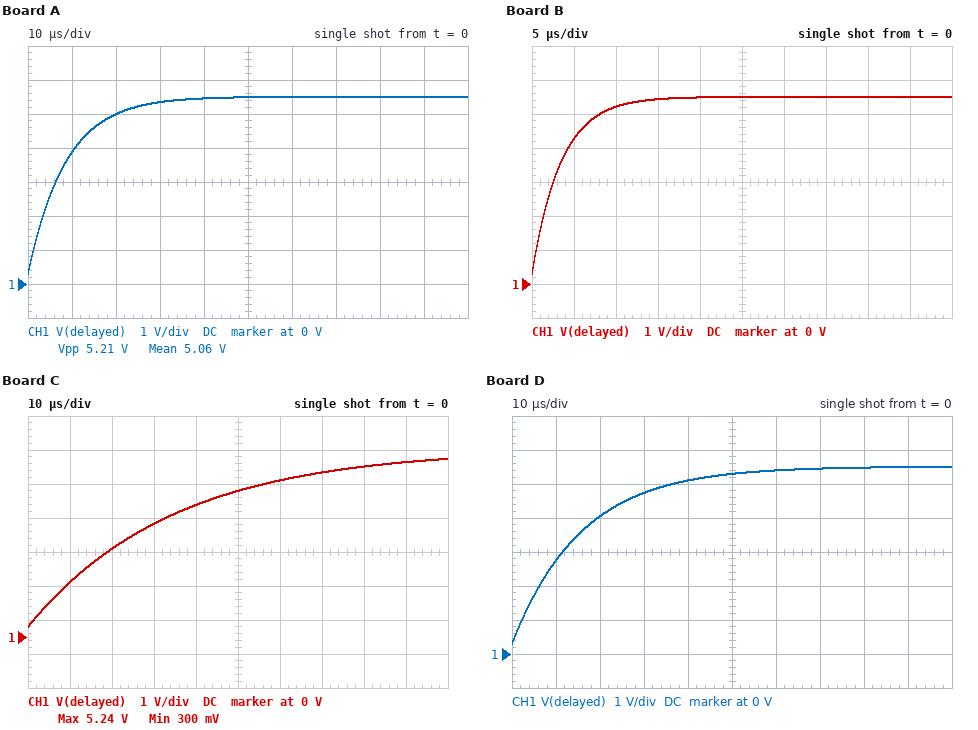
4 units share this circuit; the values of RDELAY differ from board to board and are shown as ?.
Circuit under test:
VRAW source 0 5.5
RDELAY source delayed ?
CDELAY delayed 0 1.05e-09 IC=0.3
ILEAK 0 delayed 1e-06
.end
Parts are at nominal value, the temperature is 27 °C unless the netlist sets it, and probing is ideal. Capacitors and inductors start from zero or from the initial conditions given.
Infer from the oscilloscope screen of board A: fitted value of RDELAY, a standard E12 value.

8.2 kΩ
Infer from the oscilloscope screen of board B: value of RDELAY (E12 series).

3.3 kΩ
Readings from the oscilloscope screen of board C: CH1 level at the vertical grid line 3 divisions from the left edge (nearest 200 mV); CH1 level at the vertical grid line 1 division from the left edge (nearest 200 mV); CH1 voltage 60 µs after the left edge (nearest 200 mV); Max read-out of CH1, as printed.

3.4 V
1.6 V
4.6 V
5.24 V
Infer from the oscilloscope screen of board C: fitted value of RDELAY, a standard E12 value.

33 kΩ
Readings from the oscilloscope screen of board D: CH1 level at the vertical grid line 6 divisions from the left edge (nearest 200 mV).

5.4 V
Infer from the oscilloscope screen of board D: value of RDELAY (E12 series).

15 kΩ
